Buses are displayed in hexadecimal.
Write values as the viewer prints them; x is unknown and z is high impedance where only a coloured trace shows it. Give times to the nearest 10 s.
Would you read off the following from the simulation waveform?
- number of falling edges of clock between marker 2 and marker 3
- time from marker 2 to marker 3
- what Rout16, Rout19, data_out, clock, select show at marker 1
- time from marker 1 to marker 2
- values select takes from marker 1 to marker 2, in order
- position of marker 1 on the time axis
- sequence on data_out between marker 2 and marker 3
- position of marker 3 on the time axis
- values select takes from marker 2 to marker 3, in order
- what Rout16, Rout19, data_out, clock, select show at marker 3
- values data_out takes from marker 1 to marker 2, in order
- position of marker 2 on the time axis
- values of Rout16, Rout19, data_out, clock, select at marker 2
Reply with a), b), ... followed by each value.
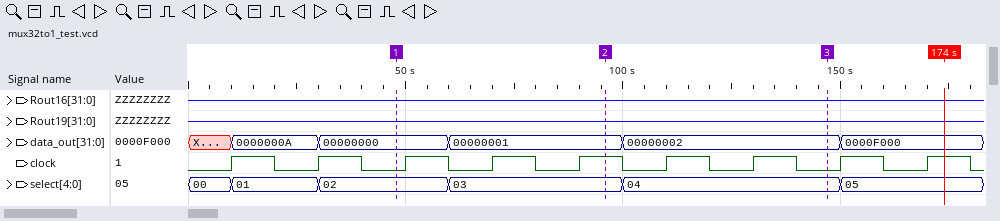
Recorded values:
a) 3
b) 50 s
c) Rout16=z, Rout19=z, data_out=00000000, clock=0, select=02
d) 50 s
e) 02, 03
f) 50 s
g) 00000001, 00000002
h) 150 s
i) 03, 04
j) Rout16=z, Rout19=z, data_out=00000002, clock=0, select=04
k) 00000000, 00000001
l) 100 s
m) Rout16=z, Rout19=z, data_out=00000001, clock=1, select=03
